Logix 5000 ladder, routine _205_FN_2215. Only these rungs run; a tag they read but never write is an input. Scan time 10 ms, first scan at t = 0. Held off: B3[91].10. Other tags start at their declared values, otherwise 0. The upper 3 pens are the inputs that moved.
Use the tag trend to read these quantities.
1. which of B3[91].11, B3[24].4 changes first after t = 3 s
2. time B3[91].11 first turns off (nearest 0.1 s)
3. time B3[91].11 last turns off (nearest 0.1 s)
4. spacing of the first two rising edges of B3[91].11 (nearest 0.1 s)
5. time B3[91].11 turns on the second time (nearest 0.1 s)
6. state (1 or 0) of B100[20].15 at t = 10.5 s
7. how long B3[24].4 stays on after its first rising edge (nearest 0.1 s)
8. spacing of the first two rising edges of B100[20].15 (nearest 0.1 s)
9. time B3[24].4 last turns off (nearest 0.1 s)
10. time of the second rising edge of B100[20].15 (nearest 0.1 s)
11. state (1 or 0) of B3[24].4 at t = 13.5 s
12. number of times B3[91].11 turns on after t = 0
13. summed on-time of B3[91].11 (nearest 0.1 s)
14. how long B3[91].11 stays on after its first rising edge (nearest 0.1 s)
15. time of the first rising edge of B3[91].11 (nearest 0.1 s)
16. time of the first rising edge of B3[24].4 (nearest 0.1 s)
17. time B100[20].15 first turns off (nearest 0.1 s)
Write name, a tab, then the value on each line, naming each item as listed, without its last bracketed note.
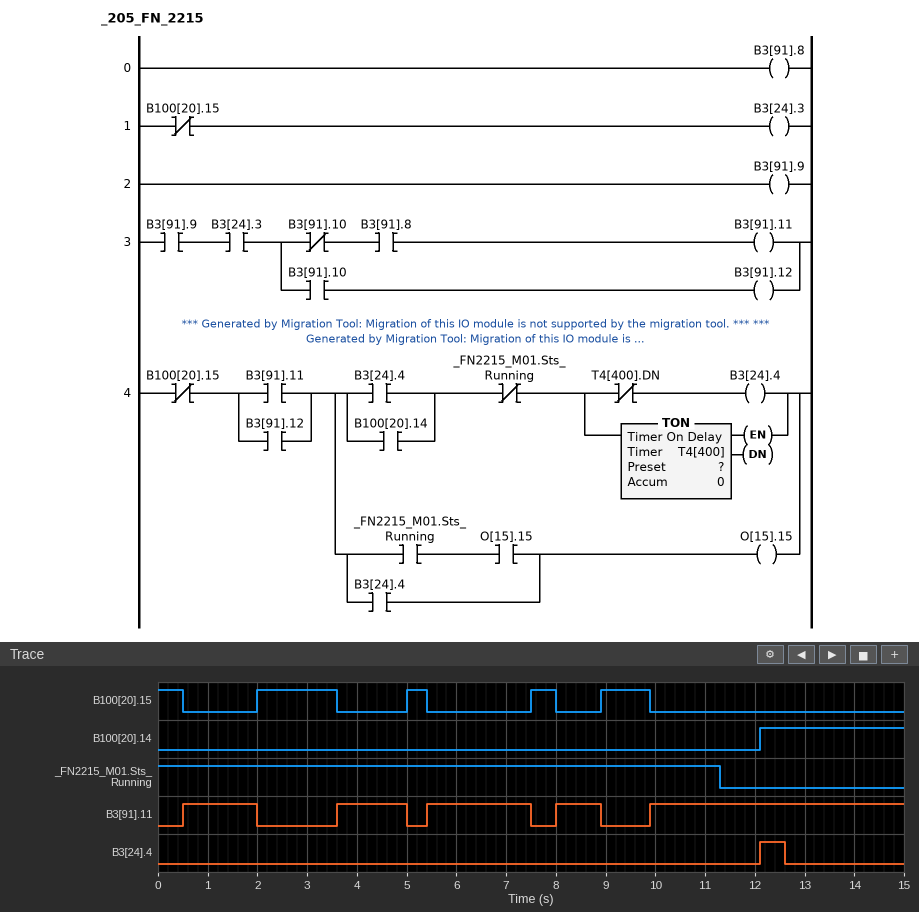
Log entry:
which of B3[91].11, B3[24].4 changes first after t = 3 s	B3[91].11
time B3[91].11 first turns off	2.0 s
time B3[91].11 last turns off	8.9 s
spacing of the first two rising edges of B3[91].11	3.1 s
time B3[91].11 turns on the second time	3.6 s
state (1 or 0) of B100[20].15 at t = 10.5 s	0
how long B3[24].4 stays on after its first rising edge	0.5 s
spacing of the first two rising edges of B100[20].15	3.0 s
time B3[24].4 last turns off	12.6 s
time of the second rising edge of B100[20].15	5.0 s
state (1 or 0) of B3[24].4 at t = 13.5 s	0
number of times B3[91].11 turns on after t = 0	5
summed on-time of B3[91].11	11.0 s
how long B3[91].11 stays on after its first rising edge	1.5 s
time of the first rising edge of B3[91].11	0.5 s
time of the first rising edge of B3[24].4	12.1 s
time B100[20].15 first turns off	0.5 s
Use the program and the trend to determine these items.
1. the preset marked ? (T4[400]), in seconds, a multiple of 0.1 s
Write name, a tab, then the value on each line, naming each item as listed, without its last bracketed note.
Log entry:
the preset marked ? (T4[400]), in seconds, a multiple of 0.1 s	0.5 s
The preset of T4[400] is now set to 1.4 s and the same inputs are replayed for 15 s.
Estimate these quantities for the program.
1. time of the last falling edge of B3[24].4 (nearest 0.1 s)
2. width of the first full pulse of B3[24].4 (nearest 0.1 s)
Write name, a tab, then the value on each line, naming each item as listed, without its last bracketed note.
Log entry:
time of the last falling edge of B3[24].4	13.5 s
width of the first full pulse of B3[24].4	1.4 s
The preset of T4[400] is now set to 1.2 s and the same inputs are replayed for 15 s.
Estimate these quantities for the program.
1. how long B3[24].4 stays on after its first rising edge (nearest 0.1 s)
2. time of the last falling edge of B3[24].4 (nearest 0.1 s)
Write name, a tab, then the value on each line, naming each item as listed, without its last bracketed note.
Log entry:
how long B3[24].4 stays on after its first rising edge	1.2 s
time of the last falling edge of B3[24].4	13.3 s
